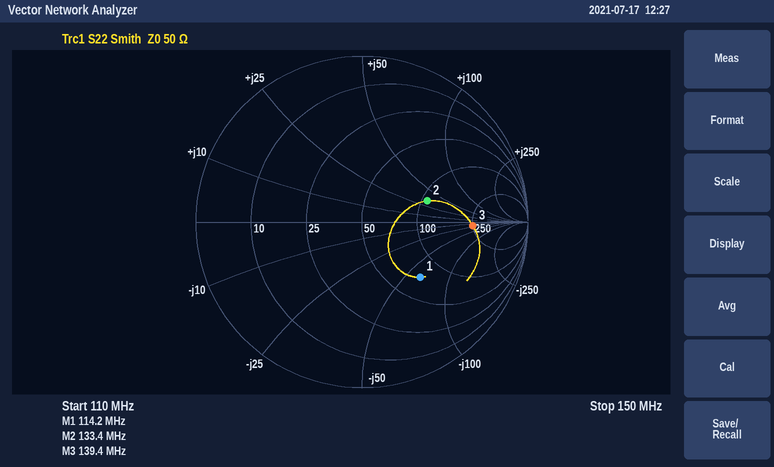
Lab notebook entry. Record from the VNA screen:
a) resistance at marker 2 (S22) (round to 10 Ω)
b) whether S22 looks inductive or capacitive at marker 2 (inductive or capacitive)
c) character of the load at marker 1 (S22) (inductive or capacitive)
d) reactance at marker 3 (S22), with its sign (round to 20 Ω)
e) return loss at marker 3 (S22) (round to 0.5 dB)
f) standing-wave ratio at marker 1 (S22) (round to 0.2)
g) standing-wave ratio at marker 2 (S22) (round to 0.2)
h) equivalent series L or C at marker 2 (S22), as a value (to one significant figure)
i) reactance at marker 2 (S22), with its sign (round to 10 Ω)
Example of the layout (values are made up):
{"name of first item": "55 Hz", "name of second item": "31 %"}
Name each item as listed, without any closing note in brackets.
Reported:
{"resistance at marker 2 (S22)": "110 Ω", "whether S22 looks inductive or capacitive at marker 2": "inductive", "character of the load at marker 1 (S22)": "capacitive", "reactance at marker 3 (S22), with its sign": "-20 Ω", "return loss at marker 3 (S22)": "3.5 dB", "standing-wave ratio at marker 1 (S22)": "2.8", "standing-wave ratio at marker 2 (S22)": "2.4", "equivalent series L or C at marker 2 (S22), as a value": "40 nH", "reactance at marker 2 (S22), with its sign": "+30 Ω"}
